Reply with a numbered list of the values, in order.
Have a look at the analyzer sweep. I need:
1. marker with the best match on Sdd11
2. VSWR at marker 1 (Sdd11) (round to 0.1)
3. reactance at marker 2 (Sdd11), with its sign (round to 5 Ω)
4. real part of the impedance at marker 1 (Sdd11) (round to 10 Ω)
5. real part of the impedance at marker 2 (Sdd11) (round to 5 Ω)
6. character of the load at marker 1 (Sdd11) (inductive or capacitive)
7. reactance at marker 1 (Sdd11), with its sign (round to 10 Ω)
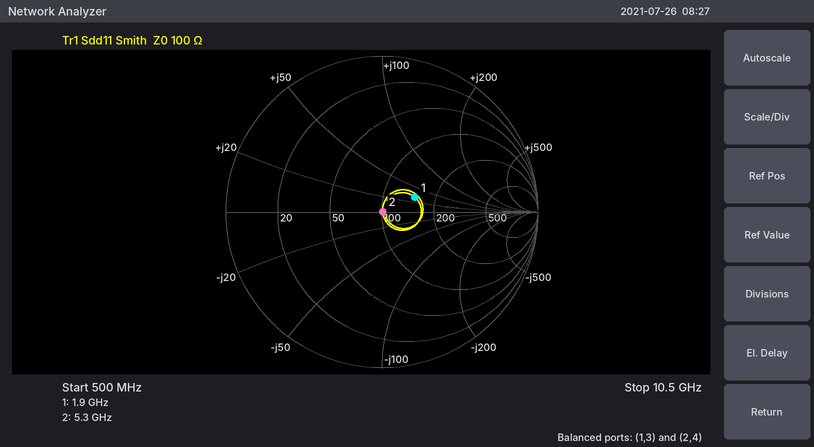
1. marker 2
2. 1.6
3. 0 Ω
4. 150 Ω
5. 100 Ω
6. inductive
7. +30 Ω
